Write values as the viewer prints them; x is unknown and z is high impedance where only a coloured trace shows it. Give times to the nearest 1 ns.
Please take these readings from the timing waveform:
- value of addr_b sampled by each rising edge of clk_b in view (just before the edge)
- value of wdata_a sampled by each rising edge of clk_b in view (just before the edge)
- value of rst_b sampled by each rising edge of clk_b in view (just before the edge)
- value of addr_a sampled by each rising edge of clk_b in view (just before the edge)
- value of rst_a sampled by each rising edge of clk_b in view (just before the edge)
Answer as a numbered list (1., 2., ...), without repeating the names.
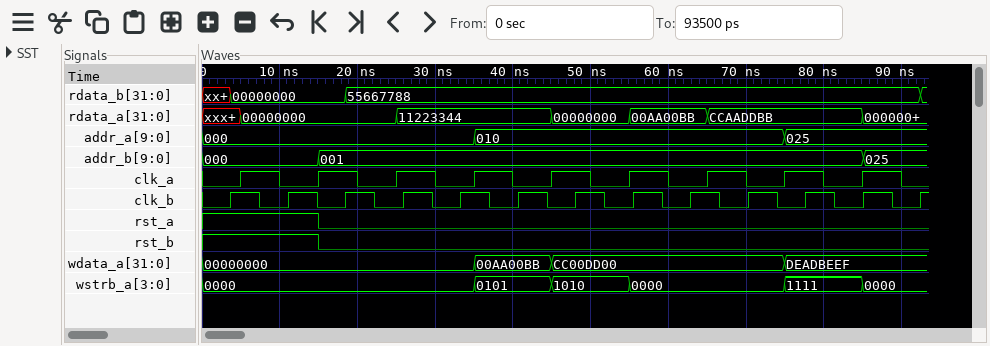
1. 000, 000, 001, 001, 001, 001, 001, 001, 001, 001, 001, 001, 025
2. 00000000, 00000000, 00000000, 00000000, 00000000, 00AA00BB, CC00DD00, CC00DD00, CC00DD00, CC00DD00, DEADBEEF, DEADBEEF, DEADBEEF
3. 1 1 0 0 0 0 0 0 0 0 0 0 0
4. 000, 000, 000, 000, 000, 010, 010, 010, 010, 010, 025, 025, 025
5. 1 1 0 0 0 0 0 0 0 0 0 0 0
